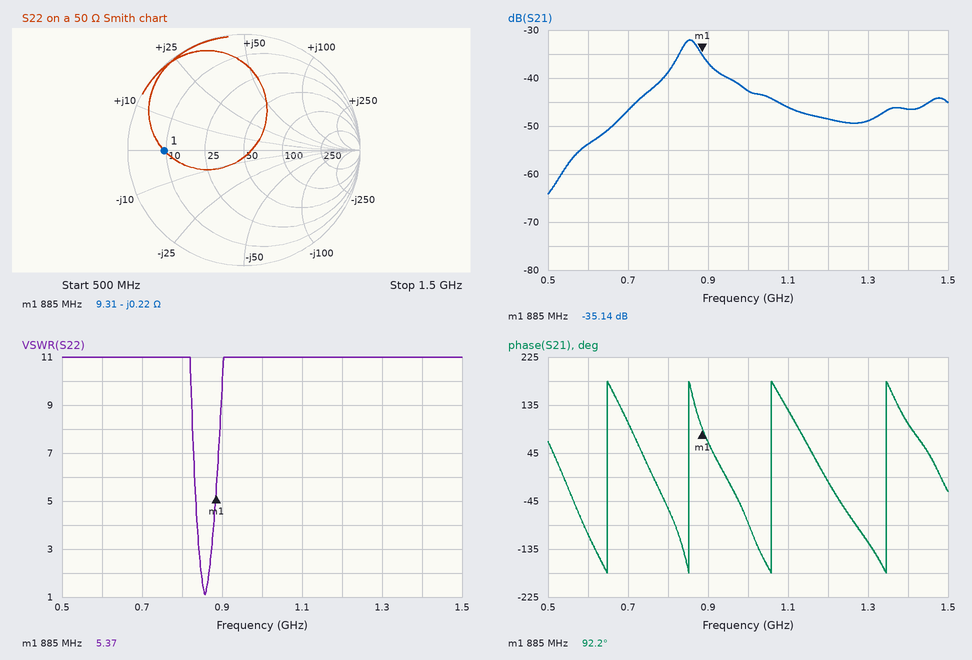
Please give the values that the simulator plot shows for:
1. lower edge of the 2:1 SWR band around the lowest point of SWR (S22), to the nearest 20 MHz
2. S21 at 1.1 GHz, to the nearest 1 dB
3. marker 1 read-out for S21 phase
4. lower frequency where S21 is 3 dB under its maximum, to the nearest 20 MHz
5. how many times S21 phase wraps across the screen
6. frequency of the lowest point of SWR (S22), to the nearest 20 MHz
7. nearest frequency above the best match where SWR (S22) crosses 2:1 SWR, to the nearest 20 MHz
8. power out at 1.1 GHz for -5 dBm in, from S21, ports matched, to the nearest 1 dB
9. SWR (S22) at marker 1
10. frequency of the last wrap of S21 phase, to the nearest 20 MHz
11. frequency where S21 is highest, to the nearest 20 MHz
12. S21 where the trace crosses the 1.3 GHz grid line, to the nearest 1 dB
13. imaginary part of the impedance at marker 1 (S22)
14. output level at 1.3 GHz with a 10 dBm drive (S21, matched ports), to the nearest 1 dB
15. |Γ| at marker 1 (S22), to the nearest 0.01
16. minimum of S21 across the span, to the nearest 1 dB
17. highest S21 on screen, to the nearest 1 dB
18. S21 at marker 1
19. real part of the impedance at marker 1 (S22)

840 MHz
-46 dB
92.2°
820 MHz
4
860 MHz
860 MHz
-51 dBm
5.37
1.34 GHz
860 MHz
-49 dB
-0.22 Ω
-39 dBm
0.69
-64 dB
-32 dB
-35.14 dB
9.31 Ω
